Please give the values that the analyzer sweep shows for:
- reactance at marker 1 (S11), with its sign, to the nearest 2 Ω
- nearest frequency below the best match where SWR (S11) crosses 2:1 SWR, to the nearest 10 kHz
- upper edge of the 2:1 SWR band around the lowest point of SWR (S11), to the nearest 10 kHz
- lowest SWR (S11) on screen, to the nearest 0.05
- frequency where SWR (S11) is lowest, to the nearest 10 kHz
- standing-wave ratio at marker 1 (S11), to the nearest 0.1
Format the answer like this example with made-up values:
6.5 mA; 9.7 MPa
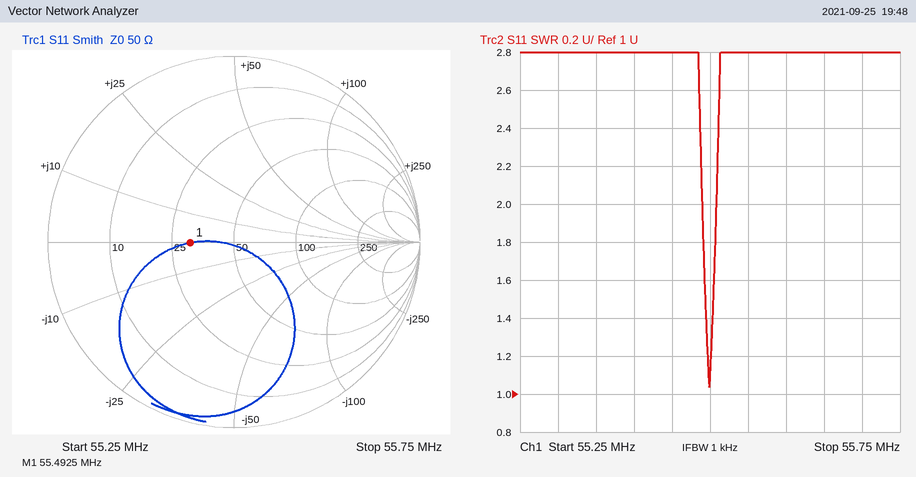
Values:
0 Ω; 55.49 MHz; 55.51 MHz; 1.05; 55.50 MHz; 1.6
